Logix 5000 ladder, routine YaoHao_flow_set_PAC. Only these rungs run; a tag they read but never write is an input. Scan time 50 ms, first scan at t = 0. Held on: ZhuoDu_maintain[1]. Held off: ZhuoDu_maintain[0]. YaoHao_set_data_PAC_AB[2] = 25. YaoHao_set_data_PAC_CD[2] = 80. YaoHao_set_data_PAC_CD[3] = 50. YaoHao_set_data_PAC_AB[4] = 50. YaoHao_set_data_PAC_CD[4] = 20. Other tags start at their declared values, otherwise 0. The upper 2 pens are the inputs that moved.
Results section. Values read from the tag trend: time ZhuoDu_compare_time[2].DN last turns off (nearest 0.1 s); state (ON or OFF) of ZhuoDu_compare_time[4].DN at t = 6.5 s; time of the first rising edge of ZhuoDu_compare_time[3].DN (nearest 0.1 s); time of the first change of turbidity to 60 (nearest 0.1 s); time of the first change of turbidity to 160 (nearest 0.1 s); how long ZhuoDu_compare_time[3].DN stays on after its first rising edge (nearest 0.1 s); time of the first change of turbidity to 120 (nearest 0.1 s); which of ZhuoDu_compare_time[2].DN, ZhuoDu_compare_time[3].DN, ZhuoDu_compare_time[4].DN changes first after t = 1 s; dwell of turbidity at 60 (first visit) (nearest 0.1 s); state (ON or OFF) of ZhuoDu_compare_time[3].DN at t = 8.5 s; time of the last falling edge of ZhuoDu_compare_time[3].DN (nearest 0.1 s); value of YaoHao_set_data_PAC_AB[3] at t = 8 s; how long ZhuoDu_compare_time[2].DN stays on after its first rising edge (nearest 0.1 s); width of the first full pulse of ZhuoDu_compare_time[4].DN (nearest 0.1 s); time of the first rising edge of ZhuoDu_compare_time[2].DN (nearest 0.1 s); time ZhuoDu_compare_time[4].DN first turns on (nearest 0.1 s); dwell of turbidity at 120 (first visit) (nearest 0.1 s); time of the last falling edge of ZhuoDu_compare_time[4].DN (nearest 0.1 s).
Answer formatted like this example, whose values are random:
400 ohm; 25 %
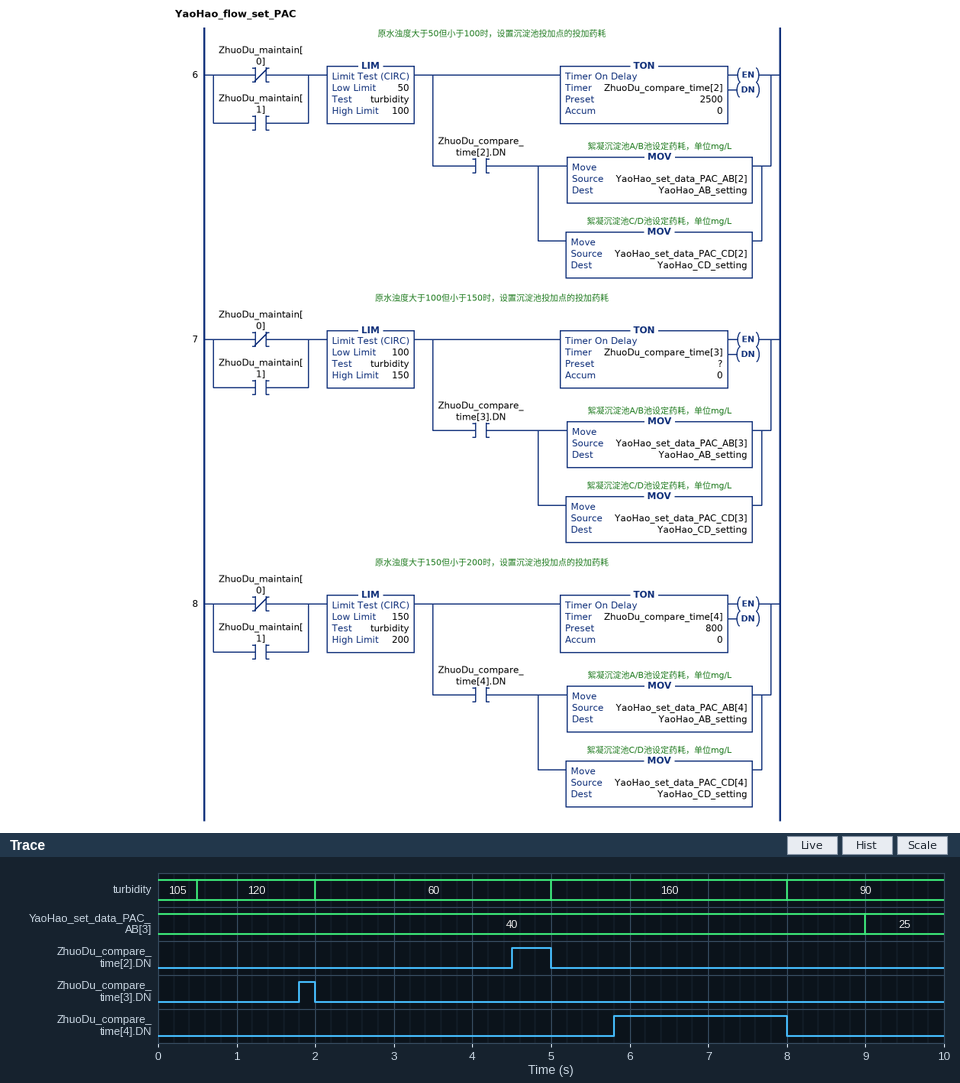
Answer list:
5.0 s; ON; 1.8 s; 2.0 s; 5.0 s; 0.2 s; 0.5 s; ZhuoDu_compare_time[3].DN; 3.0 s; OFF; 2.0 s; 40; 0.5 s; 2.2 s; 4.5 s; 5.8 s; 1.5 s; 8.0 s
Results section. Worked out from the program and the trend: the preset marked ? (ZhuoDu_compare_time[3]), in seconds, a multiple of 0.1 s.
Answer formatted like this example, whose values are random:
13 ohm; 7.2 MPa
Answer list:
1.8 s
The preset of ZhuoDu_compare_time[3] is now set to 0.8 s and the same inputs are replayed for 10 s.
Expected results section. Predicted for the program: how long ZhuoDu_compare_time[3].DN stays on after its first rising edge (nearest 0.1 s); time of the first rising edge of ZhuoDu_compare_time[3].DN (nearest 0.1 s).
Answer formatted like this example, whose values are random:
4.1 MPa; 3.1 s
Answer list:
1.2 s; 0.8 s
